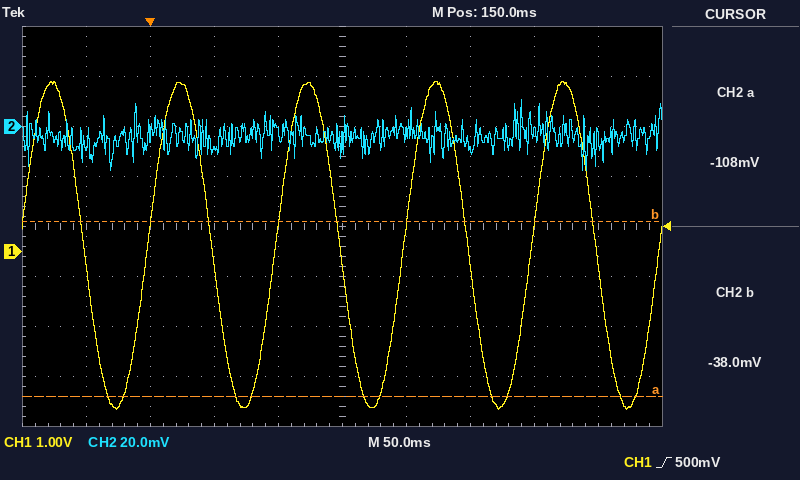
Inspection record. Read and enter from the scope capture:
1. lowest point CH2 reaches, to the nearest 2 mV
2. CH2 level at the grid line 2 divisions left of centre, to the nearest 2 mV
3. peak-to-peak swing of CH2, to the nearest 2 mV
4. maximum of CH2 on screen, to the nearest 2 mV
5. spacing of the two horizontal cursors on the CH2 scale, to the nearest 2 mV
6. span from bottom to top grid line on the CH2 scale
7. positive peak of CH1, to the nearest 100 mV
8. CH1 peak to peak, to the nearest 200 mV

-18 mV
-10 mV
28 mV
10 mV
70 mV
160 mV
3.4 V
6.6 V
